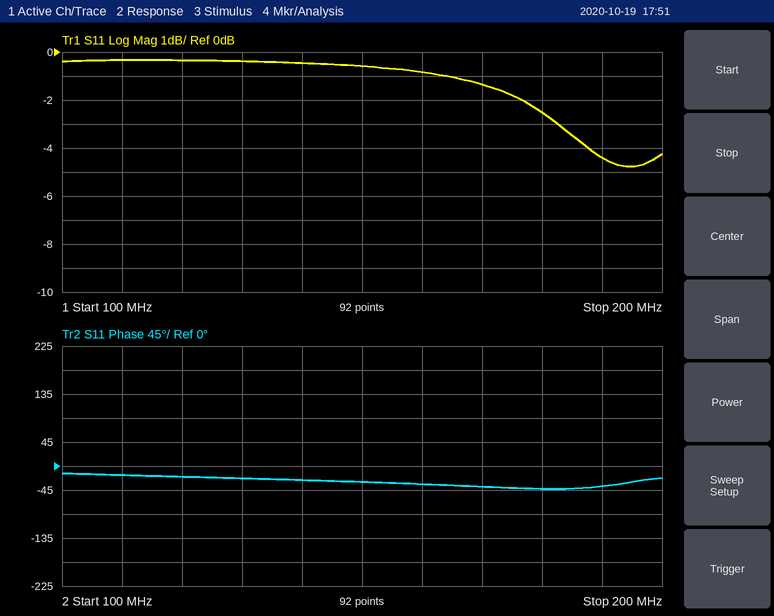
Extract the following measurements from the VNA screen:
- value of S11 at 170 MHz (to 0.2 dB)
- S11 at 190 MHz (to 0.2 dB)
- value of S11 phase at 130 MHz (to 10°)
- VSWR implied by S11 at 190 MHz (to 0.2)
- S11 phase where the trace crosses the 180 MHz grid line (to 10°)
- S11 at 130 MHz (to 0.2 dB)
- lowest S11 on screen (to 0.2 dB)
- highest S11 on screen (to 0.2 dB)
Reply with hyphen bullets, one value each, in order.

- -1.4 dB
- -4.4 dB
- -20°
- 4.0
- -40°
- -0.4 dB
- -4.8 dB
- -0.4 dB
